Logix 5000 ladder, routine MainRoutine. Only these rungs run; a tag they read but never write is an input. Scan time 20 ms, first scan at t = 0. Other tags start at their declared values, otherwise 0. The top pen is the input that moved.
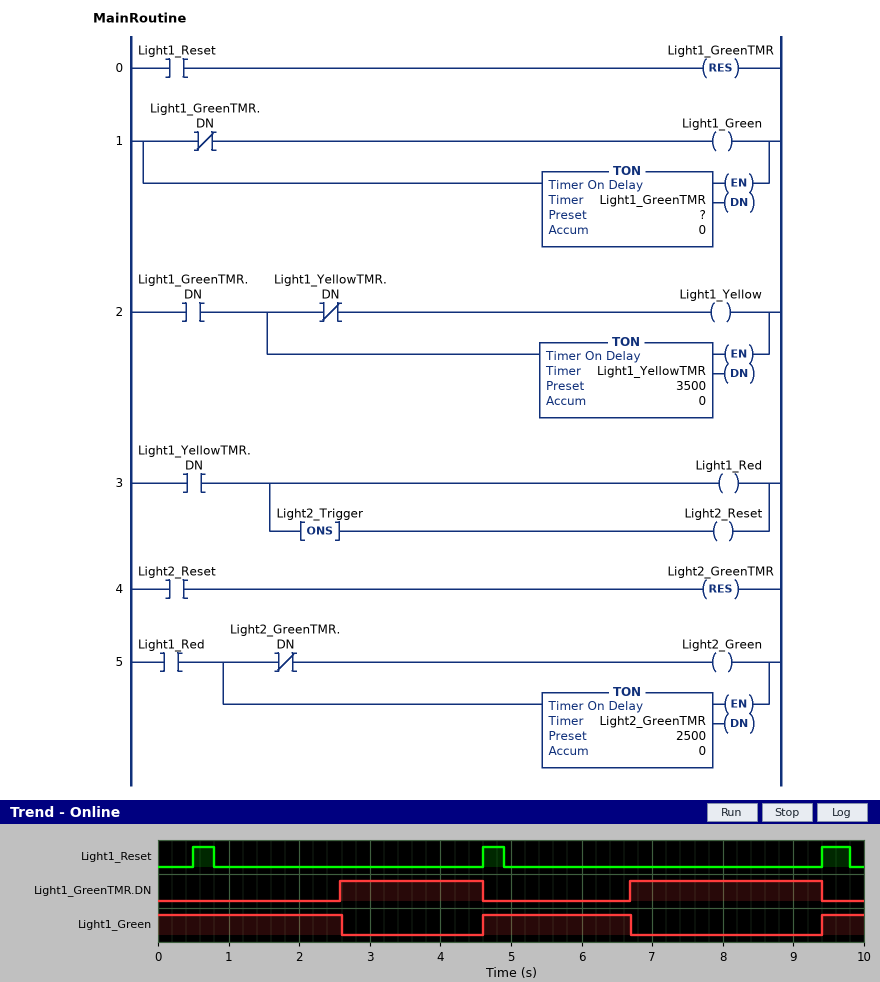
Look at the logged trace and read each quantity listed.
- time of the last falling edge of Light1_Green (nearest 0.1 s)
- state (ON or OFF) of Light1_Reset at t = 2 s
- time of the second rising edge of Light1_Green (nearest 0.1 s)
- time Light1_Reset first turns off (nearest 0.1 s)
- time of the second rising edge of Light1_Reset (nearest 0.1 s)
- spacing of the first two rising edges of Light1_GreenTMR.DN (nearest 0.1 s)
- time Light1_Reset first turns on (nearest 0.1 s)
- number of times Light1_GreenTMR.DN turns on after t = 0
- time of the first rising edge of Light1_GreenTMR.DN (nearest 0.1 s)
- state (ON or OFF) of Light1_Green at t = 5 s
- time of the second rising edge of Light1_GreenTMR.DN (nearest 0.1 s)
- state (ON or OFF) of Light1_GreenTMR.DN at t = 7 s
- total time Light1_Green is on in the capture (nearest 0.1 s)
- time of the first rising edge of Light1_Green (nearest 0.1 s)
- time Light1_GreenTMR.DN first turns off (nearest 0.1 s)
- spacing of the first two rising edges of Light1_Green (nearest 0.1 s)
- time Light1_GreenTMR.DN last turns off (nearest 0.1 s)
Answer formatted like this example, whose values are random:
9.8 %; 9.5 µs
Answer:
6.7 s; OFF; 9.4 s; 0.8 s; 4.6 s; 4.1 s; 0.5 s; 2; 2.6 s; ON; 6.7 s; ON; 5.3 s; 4.6 s; 4.6 s; 4.8 s; 9.4 s
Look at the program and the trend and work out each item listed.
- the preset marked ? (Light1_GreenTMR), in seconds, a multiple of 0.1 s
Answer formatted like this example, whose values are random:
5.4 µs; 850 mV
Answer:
1.8 s
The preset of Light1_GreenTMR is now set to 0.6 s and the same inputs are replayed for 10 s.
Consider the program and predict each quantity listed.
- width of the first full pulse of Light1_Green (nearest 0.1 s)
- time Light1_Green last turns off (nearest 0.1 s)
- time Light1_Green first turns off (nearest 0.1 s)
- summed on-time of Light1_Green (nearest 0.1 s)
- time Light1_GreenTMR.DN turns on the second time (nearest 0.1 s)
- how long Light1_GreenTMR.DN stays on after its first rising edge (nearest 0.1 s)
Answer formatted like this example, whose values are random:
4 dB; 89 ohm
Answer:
0.9 s; 5.5 s; 1.4 s; 2.9 s; 5.5 s; 3.2 s
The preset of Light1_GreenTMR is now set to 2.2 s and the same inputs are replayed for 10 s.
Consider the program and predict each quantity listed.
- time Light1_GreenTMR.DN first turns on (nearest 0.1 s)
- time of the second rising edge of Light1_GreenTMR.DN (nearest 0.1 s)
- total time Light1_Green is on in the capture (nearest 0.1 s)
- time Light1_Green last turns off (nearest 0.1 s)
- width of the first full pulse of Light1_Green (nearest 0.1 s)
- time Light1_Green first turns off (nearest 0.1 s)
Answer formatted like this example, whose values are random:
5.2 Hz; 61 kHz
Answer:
3.0 s; 7.1 s; 6.1 s; 7.1 s; 2.5 s; 3.0 s
